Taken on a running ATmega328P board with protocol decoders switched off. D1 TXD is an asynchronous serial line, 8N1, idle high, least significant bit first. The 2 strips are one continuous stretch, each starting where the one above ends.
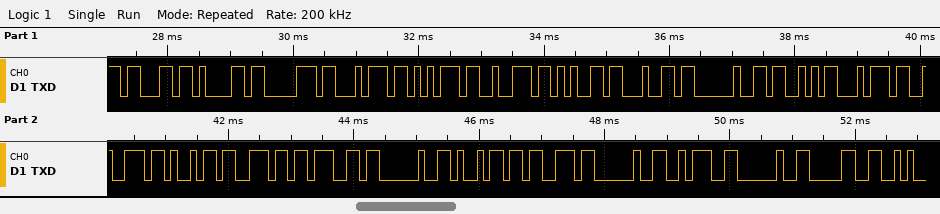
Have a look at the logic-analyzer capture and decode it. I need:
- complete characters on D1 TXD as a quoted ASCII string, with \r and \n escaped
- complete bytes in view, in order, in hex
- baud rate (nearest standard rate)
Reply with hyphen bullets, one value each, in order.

- "captured String is : 0"
- 0x63 0x61 0x70 0x74 0x75 0x72 0x65 0x64 0x20 0x53 0x74 0x72 0x69 0x6E 0x67 0x20 0x69 0x73 0x20 0x3A 0x20 0x30
- 9600 baud
